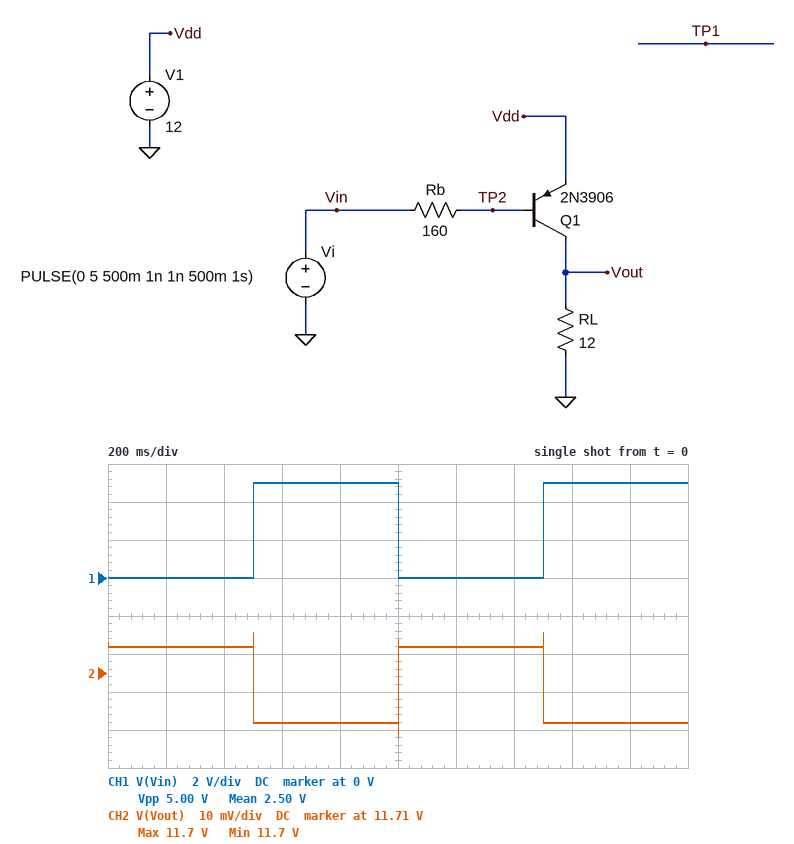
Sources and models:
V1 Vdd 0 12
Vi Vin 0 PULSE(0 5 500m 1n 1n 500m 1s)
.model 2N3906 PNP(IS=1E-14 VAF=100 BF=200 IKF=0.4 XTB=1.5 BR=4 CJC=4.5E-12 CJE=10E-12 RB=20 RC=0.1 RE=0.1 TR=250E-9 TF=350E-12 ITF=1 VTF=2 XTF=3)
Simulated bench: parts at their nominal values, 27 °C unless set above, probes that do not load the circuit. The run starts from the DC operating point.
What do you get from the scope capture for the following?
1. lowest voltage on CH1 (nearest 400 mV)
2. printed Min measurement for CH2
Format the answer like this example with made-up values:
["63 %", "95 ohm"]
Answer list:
["0 V", "11.7 V"]
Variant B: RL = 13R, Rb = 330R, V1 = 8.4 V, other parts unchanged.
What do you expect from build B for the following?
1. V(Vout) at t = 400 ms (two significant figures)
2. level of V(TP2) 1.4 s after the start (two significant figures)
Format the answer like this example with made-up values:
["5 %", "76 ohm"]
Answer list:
["8.2 V", "7.1 V"]
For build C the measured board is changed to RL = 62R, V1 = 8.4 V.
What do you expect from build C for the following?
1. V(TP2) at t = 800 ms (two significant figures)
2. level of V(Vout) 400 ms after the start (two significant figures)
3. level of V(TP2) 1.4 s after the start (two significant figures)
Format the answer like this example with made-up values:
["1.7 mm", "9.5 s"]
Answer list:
["7.3 V", "8.3 V", "6.7 V"]
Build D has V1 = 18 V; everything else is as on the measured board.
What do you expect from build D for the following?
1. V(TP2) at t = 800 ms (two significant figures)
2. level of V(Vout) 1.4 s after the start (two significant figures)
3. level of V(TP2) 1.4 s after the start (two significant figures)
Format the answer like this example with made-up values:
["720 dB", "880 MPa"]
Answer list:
["16 V", "18 V", "15 V"]
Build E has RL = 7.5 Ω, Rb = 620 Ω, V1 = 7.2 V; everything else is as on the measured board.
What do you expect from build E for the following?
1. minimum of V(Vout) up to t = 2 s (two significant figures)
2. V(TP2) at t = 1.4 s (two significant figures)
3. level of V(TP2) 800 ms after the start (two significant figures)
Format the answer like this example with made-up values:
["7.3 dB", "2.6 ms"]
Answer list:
["2.0 V", "6.1 V", "6.3 V"]
